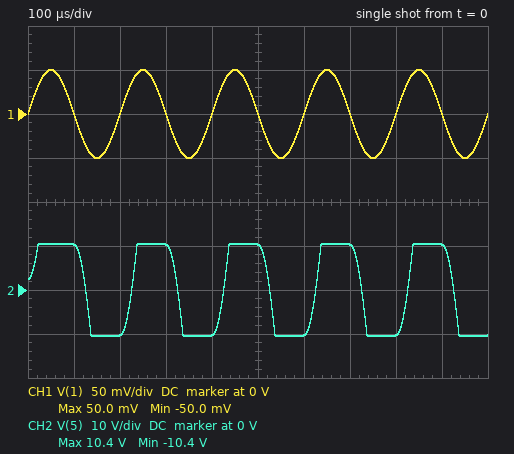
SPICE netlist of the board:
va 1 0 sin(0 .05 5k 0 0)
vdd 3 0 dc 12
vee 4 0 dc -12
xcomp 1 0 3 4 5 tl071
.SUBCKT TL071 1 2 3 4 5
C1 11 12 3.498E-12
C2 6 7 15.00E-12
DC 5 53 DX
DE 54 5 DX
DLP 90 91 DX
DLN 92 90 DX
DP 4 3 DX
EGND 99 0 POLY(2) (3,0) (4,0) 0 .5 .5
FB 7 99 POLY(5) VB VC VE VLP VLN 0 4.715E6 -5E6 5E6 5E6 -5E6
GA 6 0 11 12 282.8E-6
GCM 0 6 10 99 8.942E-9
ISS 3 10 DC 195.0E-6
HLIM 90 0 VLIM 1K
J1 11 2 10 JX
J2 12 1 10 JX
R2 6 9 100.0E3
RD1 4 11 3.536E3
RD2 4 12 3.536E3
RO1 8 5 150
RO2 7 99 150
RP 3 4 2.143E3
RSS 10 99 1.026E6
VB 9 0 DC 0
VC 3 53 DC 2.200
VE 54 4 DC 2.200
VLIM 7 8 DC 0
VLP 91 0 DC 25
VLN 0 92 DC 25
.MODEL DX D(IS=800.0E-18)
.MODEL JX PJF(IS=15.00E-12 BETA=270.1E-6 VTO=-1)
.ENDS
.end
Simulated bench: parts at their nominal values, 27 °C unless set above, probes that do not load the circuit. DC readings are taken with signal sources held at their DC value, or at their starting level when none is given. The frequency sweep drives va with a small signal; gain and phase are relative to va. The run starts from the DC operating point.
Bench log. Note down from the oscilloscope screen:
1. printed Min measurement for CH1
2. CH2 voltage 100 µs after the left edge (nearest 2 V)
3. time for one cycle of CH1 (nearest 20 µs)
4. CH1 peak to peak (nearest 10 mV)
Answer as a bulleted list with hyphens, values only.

- -50.0 mV
- 10 V
- 200 µs
- 100 mV
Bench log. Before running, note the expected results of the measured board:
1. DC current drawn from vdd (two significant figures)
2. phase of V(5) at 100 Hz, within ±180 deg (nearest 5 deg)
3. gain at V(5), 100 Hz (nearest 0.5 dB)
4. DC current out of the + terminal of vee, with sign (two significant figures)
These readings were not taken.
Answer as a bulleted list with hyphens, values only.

- 11 mA
- -80 deg
- 90.5 dB
- -11 mA
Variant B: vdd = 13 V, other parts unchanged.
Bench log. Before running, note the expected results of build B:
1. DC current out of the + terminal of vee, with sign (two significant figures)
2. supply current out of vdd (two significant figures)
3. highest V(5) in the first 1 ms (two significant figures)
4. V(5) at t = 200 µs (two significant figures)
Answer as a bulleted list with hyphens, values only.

- -12 mA
- 12 mA
- 11 V
- -10 V
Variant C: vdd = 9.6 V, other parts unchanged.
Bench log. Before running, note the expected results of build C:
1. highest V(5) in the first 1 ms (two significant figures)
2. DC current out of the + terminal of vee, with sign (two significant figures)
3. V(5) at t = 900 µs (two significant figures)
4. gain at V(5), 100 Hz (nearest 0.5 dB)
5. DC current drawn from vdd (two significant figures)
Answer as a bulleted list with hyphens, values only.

- 8.0 V
- -10 mA
- 7.9 V
- 90.5 dB
- 10 mA
